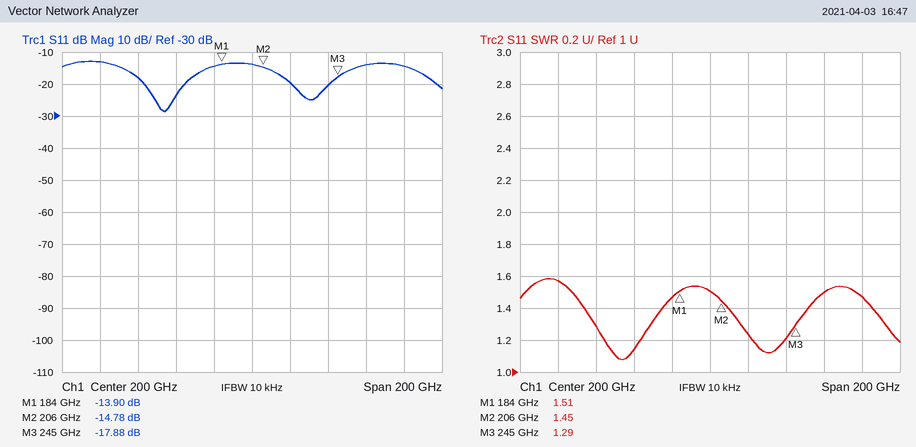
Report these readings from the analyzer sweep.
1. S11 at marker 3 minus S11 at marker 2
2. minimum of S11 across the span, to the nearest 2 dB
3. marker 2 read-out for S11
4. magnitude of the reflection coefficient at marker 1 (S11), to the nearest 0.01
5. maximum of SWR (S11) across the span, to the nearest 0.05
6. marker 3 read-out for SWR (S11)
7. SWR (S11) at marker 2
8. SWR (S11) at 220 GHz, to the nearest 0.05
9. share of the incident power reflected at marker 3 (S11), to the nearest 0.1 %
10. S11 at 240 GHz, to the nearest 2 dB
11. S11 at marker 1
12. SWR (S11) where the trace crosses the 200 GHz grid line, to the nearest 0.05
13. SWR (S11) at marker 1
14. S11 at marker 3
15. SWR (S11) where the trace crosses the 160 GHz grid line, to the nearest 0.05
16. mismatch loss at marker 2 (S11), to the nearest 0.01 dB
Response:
-3.10 dB
-28 dB
-14.78 dB
0.20
1.60
1.29
1.45
1.25
1.6 %
-20 dB
-13.90 dB
1.50
1.51
-17.88 dB
1.15
0.15 dB
